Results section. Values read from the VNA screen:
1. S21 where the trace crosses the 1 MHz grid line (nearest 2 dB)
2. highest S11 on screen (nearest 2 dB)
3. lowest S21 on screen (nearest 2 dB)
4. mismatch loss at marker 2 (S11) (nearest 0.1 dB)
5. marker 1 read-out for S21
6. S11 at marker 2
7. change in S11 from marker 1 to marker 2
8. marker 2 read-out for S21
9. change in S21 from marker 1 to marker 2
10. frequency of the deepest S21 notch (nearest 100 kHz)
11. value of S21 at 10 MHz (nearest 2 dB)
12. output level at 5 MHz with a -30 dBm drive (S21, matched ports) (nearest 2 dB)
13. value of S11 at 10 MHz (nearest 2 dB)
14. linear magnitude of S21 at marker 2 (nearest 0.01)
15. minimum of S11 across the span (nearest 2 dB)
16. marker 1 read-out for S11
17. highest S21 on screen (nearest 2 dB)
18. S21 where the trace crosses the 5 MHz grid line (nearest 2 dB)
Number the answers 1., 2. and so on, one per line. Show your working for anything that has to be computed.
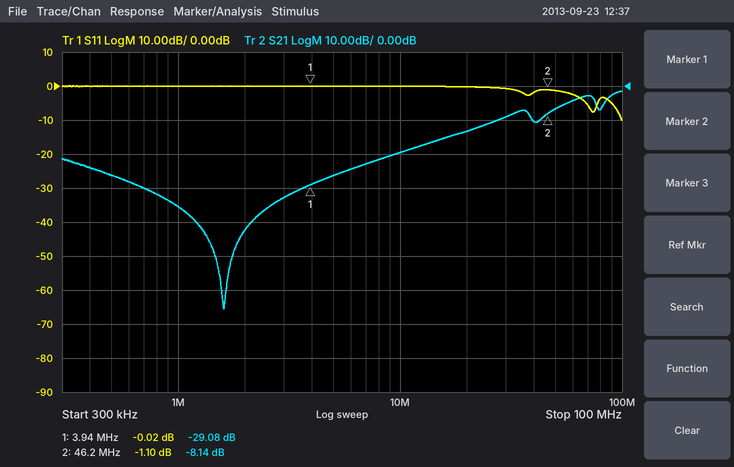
1. -36 dB
2. 0 dB
3. -66 dB
4. −10 log10(1 − 10^(-1.1/10)) ≈ 6.5 dB
5. -29.08 dB
6. -1.10 dB
7. -1.1 − (-0.02) = -1.08 dB
8. -8.14 dB
9. -8.14 − (-29.08) = 20.94 dB
10. 1.6 MHz
11. -20 dB
12. -30 dBm + (-26 dB) = -56 dBm
13. 0 dB
14. 10^(-8.14/20) ≈ 0.39
15. -10 dB
16. -0.02 dB
17. -2 dB
18. -26 dB
